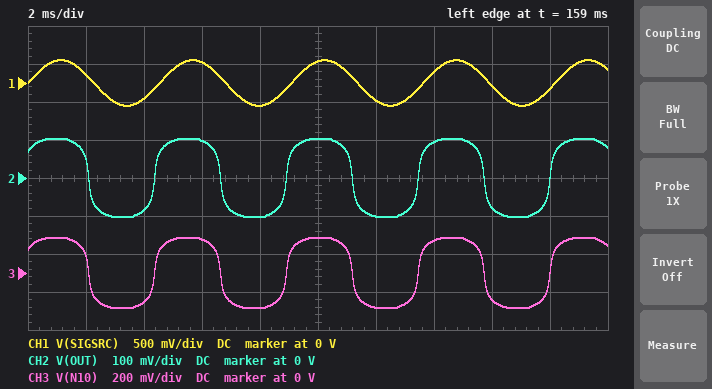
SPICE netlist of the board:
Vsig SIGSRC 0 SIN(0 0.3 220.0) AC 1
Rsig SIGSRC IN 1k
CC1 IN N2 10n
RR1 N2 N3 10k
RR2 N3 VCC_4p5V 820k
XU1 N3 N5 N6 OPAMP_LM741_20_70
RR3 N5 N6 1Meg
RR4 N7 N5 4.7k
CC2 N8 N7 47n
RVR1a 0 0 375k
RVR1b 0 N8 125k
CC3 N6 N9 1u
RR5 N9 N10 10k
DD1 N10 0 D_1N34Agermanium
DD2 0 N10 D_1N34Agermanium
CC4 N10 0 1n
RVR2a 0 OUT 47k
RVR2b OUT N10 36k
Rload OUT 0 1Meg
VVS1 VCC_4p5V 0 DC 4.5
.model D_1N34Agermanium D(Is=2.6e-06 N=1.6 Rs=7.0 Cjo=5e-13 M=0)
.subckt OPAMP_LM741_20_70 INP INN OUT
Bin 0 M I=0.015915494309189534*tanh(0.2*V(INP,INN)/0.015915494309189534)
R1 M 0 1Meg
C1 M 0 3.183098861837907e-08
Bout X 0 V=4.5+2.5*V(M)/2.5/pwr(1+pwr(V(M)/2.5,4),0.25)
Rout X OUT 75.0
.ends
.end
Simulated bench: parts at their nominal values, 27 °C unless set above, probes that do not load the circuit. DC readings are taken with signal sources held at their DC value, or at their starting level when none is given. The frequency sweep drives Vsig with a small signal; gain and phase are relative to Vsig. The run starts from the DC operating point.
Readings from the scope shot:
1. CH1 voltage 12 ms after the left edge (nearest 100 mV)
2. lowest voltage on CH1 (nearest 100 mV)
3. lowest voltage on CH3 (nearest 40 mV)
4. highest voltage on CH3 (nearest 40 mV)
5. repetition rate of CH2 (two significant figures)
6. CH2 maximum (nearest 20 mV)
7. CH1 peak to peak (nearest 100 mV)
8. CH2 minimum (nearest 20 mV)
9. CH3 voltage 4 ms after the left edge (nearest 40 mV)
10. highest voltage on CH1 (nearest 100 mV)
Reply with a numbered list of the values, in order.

1. -200 mV
2. -300 mV
3. -200 mV
4. 200 mV
5. 220 Hz
6. 100 mV
7. 600 mV
8. -100 mV
9. -160 mV
10. 300 mV
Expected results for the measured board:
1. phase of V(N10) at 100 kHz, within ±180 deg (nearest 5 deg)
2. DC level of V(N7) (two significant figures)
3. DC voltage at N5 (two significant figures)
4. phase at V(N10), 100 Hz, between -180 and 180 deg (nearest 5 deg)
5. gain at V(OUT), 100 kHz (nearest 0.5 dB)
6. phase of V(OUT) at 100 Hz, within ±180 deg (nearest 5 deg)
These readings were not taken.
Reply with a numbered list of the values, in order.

1. -110 deg
2. 4.5 V
3. 4.5 V
4. 30 deg
5. -5.5 dB
6. 30 deg
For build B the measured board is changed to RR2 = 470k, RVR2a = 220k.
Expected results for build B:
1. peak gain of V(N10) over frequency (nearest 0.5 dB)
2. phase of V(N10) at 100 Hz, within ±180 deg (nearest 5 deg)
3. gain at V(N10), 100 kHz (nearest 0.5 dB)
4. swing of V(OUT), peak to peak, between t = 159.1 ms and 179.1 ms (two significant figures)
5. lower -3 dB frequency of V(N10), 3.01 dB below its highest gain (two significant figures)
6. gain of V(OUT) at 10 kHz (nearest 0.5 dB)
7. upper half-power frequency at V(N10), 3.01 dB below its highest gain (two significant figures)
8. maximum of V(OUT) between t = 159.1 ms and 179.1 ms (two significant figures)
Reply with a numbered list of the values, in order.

1. 11.5 dB
2. 35 deg
3. -0.5 dB
4. 310 mV
5. 47 Hz
6. 9.5 dB
7. 34 kHz
8. 160 mV
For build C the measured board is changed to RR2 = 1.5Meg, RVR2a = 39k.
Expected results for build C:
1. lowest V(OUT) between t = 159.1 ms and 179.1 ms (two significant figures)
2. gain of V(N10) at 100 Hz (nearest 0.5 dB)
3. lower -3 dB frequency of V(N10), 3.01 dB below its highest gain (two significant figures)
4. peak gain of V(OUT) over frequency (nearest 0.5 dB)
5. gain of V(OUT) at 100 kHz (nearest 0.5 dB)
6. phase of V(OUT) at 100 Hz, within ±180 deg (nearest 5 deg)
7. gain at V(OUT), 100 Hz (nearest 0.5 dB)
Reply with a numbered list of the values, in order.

1. -95 mV
2. 11.0 dB
3. 32 Hz
4. 5.5 dB
5. -6.0 dB
6. 25 deg
7. 5.0 dB
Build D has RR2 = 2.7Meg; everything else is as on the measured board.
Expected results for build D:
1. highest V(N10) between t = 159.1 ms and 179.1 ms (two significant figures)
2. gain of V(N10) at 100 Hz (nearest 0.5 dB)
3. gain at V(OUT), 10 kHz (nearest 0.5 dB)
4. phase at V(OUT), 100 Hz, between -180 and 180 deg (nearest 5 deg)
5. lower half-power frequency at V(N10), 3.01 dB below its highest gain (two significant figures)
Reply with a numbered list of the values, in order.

1. 190 mV
2. 11.0 dB
3. 6.0 dB
4. 20 deg
5. 30 Hz
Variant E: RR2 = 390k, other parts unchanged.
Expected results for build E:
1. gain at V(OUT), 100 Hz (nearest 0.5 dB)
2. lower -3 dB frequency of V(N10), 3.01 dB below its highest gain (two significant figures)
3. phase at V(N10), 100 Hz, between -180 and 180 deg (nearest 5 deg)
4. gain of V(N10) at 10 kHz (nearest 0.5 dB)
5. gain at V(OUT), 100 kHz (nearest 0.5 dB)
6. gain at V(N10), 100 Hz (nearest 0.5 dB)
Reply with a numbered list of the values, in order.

1. 5.0 dB
2. 53 Hz
3. 40 deg
4. 10.5 dB
5. -5.5 dB
6. 10.0 dB
